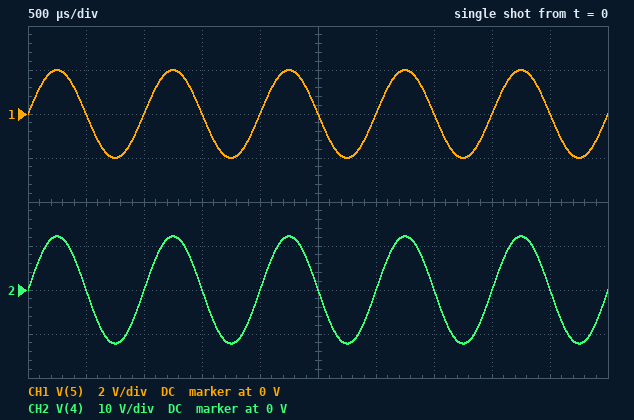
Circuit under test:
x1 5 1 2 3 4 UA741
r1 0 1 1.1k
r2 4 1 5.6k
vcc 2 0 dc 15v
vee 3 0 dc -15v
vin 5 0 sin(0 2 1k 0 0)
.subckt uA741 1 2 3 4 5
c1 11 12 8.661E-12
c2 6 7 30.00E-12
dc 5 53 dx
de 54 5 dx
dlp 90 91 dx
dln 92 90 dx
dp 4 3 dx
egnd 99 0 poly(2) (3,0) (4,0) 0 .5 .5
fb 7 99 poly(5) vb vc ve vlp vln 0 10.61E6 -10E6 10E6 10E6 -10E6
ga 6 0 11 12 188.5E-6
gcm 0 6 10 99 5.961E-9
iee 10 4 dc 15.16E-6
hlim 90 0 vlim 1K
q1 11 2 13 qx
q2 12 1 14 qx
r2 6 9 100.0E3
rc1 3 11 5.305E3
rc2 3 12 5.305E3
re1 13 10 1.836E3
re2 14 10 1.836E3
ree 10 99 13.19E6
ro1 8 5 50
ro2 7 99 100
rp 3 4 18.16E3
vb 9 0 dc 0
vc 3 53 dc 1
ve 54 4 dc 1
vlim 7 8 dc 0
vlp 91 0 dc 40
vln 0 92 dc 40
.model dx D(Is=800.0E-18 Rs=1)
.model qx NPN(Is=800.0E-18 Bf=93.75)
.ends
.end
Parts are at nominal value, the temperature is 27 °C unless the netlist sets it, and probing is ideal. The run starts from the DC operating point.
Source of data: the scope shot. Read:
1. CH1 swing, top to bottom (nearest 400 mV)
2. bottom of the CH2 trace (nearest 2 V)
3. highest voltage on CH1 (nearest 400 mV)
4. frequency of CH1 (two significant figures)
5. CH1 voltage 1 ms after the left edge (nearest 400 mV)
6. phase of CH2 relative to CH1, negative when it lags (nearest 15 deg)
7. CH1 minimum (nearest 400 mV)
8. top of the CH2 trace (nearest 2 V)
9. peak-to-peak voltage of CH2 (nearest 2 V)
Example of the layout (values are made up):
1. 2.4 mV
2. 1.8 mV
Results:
1. 4.0 V
2. -12 V
3. 2.0 V
4. 1.0 kHz
5. 0 V
6. 0 deg
7. -2.0 V
8. 12 V
9. 24 V
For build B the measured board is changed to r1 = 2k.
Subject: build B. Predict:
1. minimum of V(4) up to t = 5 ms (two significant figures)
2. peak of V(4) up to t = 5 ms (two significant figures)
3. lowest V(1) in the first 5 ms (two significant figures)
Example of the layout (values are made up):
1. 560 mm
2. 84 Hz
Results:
1. -7.6 V
2. 7.6 V
3. -2.0 V
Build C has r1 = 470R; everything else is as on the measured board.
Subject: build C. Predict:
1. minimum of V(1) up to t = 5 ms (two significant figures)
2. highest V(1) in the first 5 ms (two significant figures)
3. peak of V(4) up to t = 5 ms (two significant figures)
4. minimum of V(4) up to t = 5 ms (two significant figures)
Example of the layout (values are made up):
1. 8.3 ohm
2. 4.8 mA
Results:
1. -1.1 V
2. 1.1 V
3. 15 V
4. -15 V
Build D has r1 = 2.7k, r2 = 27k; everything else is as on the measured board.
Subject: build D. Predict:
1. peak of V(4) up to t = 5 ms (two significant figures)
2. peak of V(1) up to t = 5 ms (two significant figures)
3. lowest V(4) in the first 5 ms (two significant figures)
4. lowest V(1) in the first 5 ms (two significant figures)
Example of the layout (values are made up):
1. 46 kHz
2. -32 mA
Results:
1. 15 V
2. 1.3 V
3. -15 V
4. -1.3 V
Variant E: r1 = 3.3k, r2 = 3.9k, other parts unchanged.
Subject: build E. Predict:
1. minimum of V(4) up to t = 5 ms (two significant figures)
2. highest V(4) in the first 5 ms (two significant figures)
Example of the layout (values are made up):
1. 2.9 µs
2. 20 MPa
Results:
1. -4.4 V
2. 4.4 V
